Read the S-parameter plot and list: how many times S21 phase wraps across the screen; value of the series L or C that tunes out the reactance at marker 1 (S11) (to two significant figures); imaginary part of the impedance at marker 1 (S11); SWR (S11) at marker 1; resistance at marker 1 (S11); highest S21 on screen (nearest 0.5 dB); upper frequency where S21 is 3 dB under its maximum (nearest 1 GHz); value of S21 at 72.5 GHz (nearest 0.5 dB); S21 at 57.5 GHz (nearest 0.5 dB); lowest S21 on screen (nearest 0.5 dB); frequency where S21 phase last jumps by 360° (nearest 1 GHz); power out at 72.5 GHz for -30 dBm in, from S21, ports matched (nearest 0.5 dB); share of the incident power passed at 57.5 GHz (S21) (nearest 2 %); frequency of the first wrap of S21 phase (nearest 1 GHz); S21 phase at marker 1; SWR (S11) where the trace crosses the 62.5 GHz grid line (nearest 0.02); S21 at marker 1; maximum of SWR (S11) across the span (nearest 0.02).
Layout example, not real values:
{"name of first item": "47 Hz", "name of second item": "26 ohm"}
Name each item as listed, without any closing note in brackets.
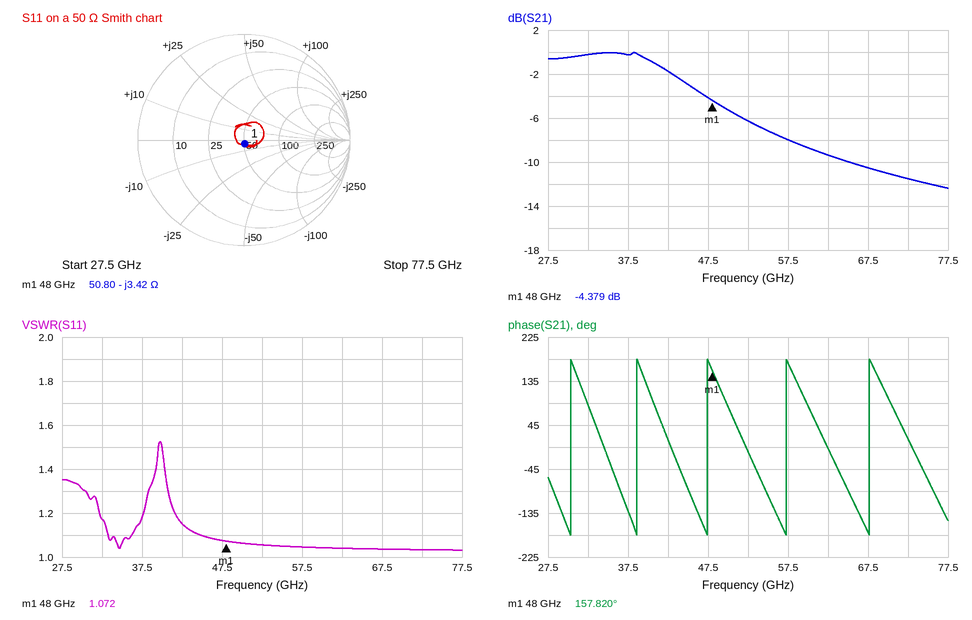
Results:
{"how many times S21 phase wraps across the screen": "5", "value of the series L or C that tunes out the reactance at marker 1 (S11)": "11 pH", "imaginary part of the impedance at marker 1": "-3.42 Ω", "SWR (S11) at marker 1": "1.072", "resistance at marker 1": "50.80 Ω", "highest S21 on screen": "0.0 dB", "upper frequency where S21 is 3 dB under its maximum": "45 GHz", "value of S21 at 72.5 GHz": "-11.5 dB", "S21 at 57.5 GHz": "-8.0 dB", "lowest S21 on screen": "-12.5 dB", "frequency where S21 phase last jumps by 360°": "68 GHz", "power out at 72.5 GHz for -30 dBm in, from S21, ports matched": "-41.5 dBm", "share of the incident power passed at 57.5 GHz (S21)": "16 %", "frequency of the first wrap of S21 phase": "30 GHz", "S21 phase at marker 1": "157.820°", "SWR (S11) where the trace crosses the 62.5 GHz grid line": "1.04", "S21 at marker 1": "-4.379 dB", "maximum of SWR (S11) across the span": "1.52"}
